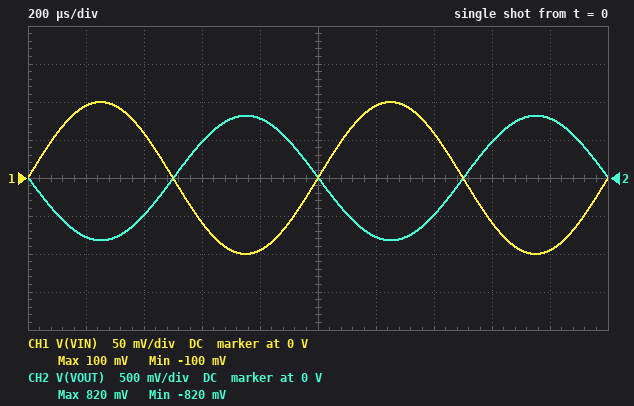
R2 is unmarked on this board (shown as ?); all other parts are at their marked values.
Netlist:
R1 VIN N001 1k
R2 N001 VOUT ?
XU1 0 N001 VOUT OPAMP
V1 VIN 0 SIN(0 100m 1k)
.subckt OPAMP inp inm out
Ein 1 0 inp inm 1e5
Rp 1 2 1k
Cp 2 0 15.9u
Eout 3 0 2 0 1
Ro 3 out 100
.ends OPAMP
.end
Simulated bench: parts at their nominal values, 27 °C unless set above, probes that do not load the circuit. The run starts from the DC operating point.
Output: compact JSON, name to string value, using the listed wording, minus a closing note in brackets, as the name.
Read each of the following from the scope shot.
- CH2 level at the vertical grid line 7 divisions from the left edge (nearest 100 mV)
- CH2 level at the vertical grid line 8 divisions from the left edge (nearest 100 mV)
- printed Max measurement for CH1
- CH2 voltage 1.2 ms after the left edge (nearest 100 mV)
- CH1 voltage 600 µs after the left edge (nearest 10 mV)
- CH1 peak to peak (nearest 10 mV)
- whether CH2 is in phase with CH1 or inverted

{"CH2 level at the vertical grid line 7 divisions from the left edge": "-500 mV", "CH2 level at the vertical grid line 8 divisions from the left edge": "500 mV", "printed Max measurement for CH1": "100 mV", "CH2 voltage 1.2 ms after the left edge": "-800 mV", "CH1 voltage 600 µs after the left edge": "-60 mV", "CH1 peak to peak": "200 mV", "whether CH2 is in phase with CH1 or inverted": "inverted"}
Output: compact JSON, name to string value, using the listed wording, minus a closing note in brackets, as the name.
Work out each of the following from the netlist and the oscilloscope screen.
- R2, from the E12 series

{"R2, from the E12 series": "8.2 kΩ"}
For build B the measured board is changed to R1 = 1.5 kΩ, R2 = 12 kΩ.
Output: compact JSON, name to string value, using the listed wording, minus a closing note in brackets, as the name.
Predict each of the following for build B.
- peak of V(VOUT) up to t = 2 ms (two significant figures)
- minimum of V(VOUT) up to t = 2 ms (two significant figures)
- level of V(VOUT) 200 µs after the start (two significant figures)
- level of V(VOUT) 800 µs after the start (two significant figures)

{"peak of V(VOUT) up to t = 2 ms": "800 mV", "minimum of V(VOUT) up to t = 2 ms": "-800 mV", "level of V(VOUT) 200 µs after the start": "-760 mV", "level of V(VOUT) 800 µs after the start": "760 mV"}
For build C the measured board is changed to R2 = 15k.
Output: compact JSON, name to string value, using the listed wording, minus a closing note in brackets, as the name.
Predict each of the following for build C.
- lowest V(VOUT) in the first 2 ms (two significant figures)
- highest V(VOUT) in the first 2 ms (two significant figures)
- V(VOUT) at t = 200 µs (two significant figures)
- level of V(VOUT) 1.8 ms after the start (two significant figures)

{"lowest V(VOUT) in the first 2 ms": "-1.5 V", "highest V(VOUT) in the first 2 ms": "1.5 V", "V(VOUT) at t = 200 µs": "-1.4 V", "level of V(VOUT) 1.8 ms after the start": "1.4 V"}
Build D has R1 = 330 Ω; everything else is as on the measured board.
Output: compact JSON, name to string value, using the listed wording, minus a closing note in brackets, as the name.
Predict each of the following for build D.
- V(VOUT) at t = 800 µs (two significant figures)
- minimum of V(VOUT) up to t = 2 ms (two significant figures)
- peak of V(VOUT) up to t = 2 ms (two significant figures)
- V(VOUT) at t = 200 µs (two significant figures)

{"V(VOUT) at t = 800 µs": "2.4 V", "minimum of V(VOUT) up to t = 2 ms": "-2.5 V", "peak of V(VOUT) up to t = 2 ms": "2.5 V", "V(VOUT) at t = 200 µs": "-2.3 V"}
